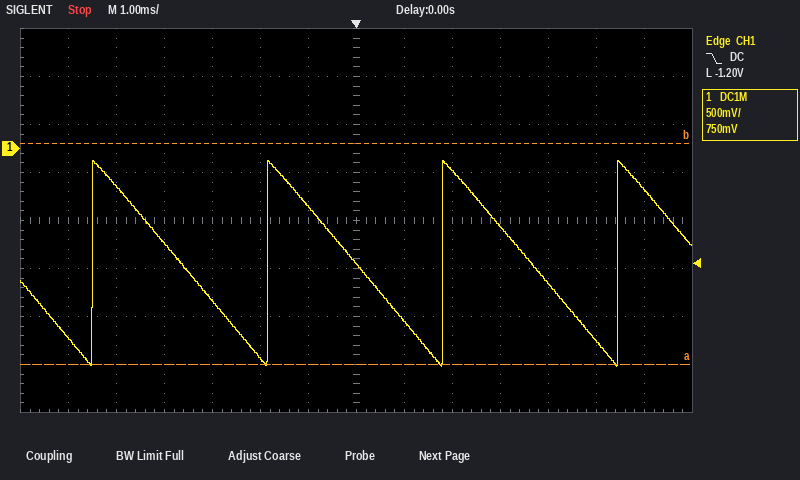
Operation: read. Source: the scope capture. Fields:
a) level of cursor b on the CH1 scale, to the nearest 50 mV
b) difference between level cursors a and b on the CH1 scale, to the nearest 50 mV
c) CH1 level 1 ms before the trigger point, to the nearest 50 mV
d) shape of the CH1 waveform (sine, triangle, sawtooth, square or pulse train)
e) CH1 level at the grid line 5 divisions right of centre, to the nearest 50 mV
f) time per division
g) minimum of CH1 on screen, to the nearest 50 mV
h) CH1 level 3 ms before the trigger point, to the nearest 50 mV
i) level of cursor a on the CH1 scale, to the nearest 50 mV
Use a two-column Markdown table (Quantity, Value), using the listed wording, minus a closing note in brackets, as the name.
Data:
| Quantity | Value |
|---|---|
| level of cursor b on the CH1 scale, to the nearest 50 mV | 50 mV |
| difference between level cursors a and b on the CH1 scale, to the nearest 50 mV | 2.30 V |
| CH1 level 1 ms before the trigger point, to the nearest 50 mV | -600 mV |
| shape of the CH1 waveform | sawtooth |
| CH1 level at the grid line 5 divisions right of centre, to the nearest 50 mV | -2.00 V |
| time per division | 1 ms |
| minimum of CH1 on screen, to the nearest 50 mV | -2.25 V |
| CH1 level 3 ms before the trigger point, to the nearest 50 mV | -1.60 V |
| level of cursor a on the CH1 scale, to the nearest 50 mV | -2.25 V |
